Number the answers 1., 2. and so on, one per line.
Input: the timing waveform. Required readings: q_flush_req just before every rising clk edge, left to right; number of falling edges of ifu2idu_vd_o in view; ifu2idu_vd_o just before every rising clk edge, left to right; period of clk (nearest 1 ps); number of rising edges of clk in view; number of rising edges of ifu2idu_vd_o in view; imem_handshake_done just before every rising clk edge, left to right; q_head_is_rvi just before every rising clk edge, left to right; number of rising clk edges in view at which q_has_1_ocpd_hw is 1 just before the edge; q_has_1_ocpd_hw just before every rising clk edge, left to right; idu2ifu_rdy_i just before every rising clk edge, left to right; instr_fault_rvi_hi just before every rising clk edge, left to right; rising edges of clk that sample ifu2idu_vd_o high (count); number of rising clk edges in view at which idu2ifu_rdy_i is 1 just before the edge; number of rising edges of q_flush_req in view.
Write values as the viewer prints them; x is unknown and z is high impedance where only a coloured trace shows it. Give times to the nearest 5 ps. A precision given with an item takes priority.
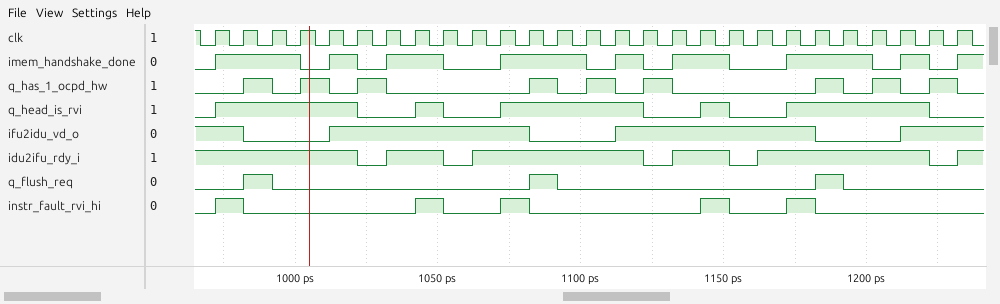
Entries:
1. 0 0 1 0 0 0 0 0 0 0 0 0 1 0 0 0 0 0 0 0 0 0 1 0 0 0 0
2. 3
3. 1 1 0 0 0 1 1 1 1 1 1 1 0 0 0 1 1 1 1 1 1 1 0 0 0 1 1
4. 10 ps
5. 27
6. 3
7. 0 1 1 1 0 1 0 1 1 0 0 1 1 1 0 1 0 1 1 0 0 1 1 1 0 1 0
8. 0 1 1 1 1 1 0 0 1 0 0 1 1 1 1 1 0 0 1 0 0 1 1 1 1 1 0
9. 9
10. 0 0 1 0 1 0 1 0 0 0 0 0 1 0 1 0 1 0 0 0 0 0 1 0 1 0 1
11. 1 1 1 1 1 1 0 1 1 0 1 1 1 1 1 1 0 1 1 0 1 1 1 1 1 1 0
12. 0 1 0 0 0 0 0 0 1 0 0 1 0 0 0 0 0 0 1 0 0 1 0 0 0 0 0
13. 18
14. 22
15. 3
